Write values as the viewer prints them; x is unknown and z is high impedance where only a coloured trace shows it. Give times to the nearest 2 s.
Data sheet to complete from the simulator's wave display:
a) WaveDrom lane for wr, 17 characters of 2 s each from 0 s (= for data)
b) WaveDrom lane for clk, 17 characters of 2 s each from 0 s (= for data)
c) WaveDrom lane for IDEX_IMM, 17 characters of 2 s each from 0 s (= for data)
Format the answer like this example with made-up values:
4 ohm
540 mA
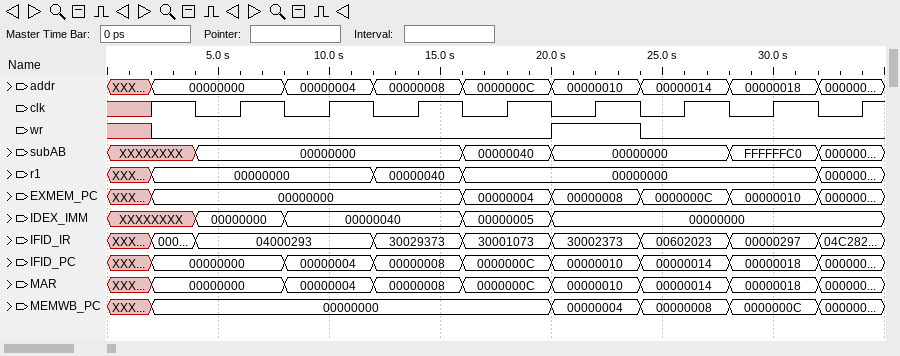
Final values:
{name: 'wr', wave: 'x0........1.0....'}
{name: 'clk', wave: 'x1010101010101010'}
{name: 'IDEX_IMM', wave: 'x.=.=...=.=......', data: '00000000 00000040 00000005 00000000'}
